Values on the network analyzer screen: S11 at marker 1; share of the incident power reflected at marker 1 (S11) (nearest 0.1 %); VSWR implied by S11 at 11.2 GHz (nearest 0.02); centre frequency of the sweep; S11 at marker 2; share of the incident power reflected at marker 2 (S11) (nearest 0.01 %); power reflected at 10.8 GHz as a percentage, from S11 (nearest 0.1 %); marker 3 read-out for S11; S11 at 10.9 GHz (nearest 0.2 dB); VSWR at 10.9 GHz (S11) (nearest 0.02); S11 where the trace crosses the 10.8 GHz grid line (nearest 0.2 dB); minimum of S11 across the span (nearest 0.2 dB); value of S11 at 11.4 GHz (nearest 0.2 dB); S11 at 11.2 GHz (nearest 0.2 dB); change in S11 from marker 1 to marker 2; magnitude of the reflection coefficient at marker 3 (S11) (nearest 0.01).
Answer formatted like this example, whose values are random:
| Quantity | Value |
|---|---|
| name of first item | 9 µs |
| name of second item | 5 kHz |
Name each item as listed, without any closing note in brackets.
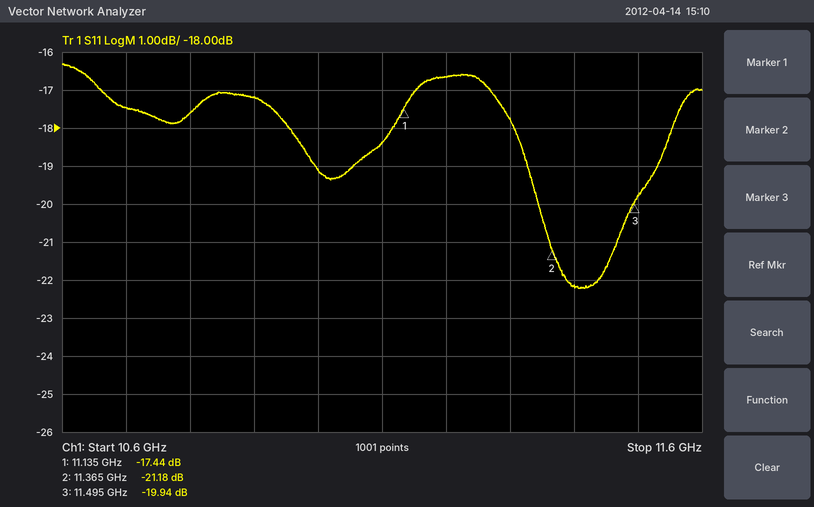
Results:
| Quantity | Value |
|---|---|
| S11 at marker 1 | -17.44 dB |
| share of the incident power reflected at marker 1 (S11) | 1.8 % |
| VSWR implied by S11 at 11.2 GHz | 1.34 |
| centre frequency of the sweep | 11.1 GHz |
| S11 at marker 2 | -21.18 dB |
| share of the incident power reflected at marker 2 (S11) | 0.76 % |
| power reflected at 10.8 GHz as a percentage, from S11 | 1.7 % |
| marker 3 read-out for S11 | -19.94 dB |
| S11 at 10.9 GHz | -17.2 dB |
| VSWR at 10.9 GHz (S11) | 1.32 |
| S11 where the trace crosses the 10.8 GHz grid line | -17.6 dB |
| minimum of S11 across the span | -22.2 dB |
| value of S11 at 11.4 GHz | -22.2 dB |
| S11 at 11.2 GHz | -16.6 dB |
| change in S11 from marker 1 to marker 2 | -3.74 dB |
| magnitude of the reflection coefficient at marker 3 (S11) | 0.10 |
